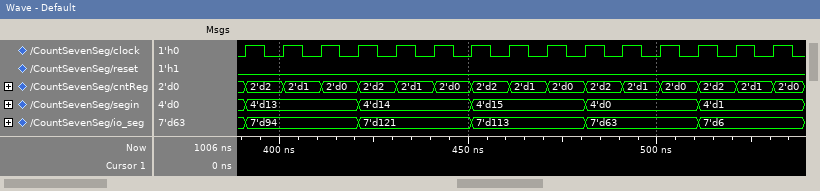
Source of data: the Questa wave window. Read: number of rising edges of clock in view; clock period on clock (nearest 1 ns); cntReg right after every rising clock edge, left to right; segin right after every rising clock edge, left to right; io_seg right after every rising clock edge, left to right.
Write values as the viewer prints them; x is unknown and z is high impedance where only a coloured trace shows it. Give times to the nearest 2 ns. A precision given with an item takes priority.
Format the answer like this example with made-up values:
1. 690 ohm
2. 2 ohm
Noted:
1. 15
2. 10 ns
3. 2'd2, 2'd1, 2'd0, 2'd2, 2'd1, 2'd0, 2'd2, 2'd1, 2'd0, 2'd2, 2'd1, 2'd0, 2'd2, 2'd1, 2'd0
4. 4'd13, 4'd13, 4'd13, 4'd14, 4'd14, 4'd14, 4'd15, 4'd15, 4'd15, 4'd0, 4'd0, 4'd0, 4'd1, 4'd1, 4'd1
5. 7'd94, 7'd94, 7'd94, 7'd121, 7'd121, 7'd121, 7'd113, 7'd113, 7'd113, 7'd63, 7'd63, 7'd63, 7'd6, 7'd6, 7'd6
